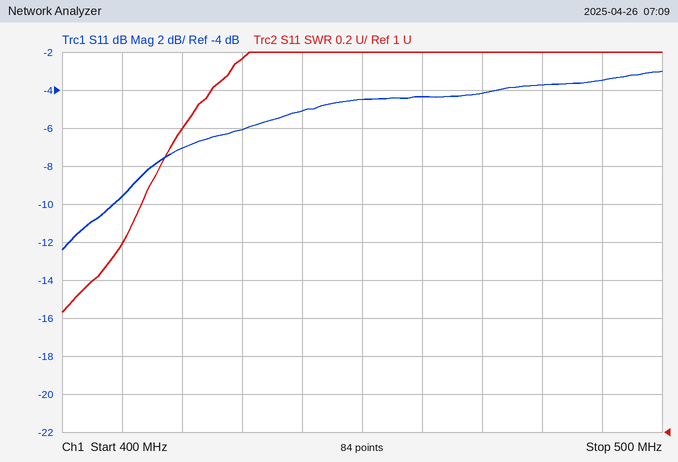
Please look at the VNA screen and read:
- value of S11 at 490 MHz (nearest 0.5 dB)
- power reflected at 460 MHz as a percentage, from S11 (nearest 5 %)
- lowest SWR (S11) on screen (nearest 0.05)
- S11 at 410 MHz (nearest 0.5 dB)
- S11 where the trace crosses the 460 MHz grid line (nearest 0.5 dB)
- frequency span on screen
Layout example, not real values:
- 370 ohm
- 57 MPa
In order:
- -3.5 dB
- 35 %
- 1.65
- -9.5 dB
- -4.5 dB
- 100 MHz
